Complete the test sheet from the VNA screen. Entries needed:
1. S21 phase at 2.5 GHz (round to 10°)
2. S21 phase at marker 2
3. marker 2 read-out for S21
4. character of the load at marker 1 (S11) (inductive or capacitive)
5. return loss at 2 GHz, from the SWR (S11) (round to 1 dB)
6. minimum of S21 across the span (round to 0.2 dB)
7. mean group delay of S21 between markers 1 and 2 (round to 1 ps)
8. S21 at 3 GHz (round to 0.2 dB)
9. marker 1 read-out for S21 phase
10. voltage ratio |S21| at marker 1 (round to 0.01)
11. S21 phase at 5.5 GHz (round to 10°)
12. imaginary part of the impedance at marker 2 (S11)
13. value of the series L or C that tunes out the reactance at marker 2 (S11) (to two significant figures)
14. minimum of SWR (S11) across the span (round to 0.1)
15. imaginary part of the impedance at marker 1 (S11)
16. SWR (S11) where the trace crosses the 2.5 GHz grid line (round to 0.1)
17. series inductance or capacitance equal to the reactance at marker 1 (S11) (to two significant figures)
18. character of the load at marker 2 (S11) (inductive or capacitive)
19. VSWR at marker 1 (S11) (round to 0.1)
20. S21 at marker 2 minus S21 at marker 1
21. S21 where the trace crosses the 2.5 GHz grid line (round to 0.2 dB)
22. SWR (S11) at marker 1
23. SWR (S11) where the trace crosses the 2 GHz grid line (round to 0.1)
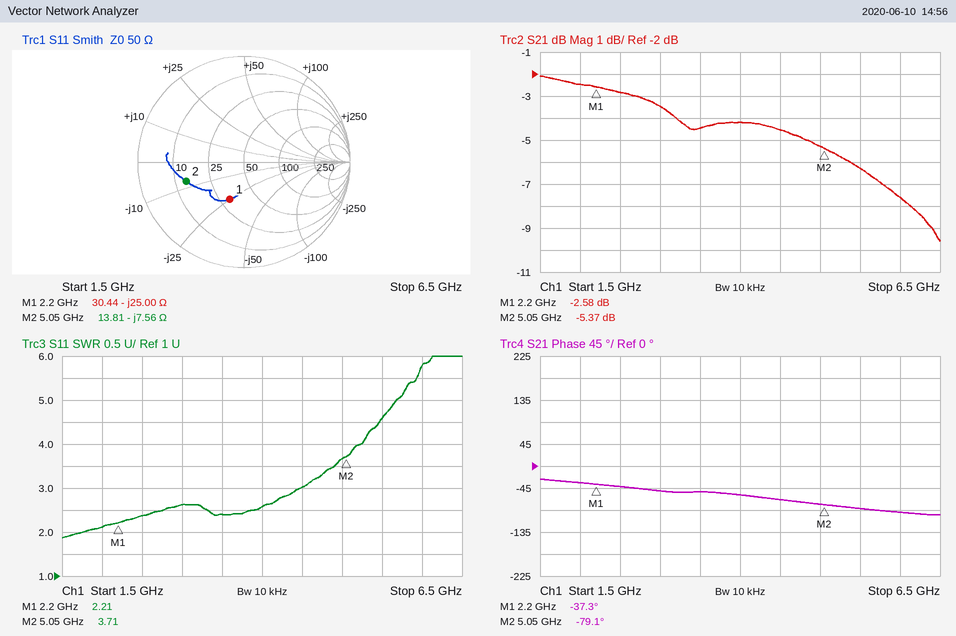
-40°
-79.1°
-5.37 dB
capacitive
9 dB
-9.6 dB
41 ps
-3.4 dB
-37.3°
0.74
-90°
-7.56 Ω
240 pH
1.9
-25.00 Ω
2.4
2.9 pF
capacitive
2.2
-2.79 dB
-2.8 dB
2.21
2.1
